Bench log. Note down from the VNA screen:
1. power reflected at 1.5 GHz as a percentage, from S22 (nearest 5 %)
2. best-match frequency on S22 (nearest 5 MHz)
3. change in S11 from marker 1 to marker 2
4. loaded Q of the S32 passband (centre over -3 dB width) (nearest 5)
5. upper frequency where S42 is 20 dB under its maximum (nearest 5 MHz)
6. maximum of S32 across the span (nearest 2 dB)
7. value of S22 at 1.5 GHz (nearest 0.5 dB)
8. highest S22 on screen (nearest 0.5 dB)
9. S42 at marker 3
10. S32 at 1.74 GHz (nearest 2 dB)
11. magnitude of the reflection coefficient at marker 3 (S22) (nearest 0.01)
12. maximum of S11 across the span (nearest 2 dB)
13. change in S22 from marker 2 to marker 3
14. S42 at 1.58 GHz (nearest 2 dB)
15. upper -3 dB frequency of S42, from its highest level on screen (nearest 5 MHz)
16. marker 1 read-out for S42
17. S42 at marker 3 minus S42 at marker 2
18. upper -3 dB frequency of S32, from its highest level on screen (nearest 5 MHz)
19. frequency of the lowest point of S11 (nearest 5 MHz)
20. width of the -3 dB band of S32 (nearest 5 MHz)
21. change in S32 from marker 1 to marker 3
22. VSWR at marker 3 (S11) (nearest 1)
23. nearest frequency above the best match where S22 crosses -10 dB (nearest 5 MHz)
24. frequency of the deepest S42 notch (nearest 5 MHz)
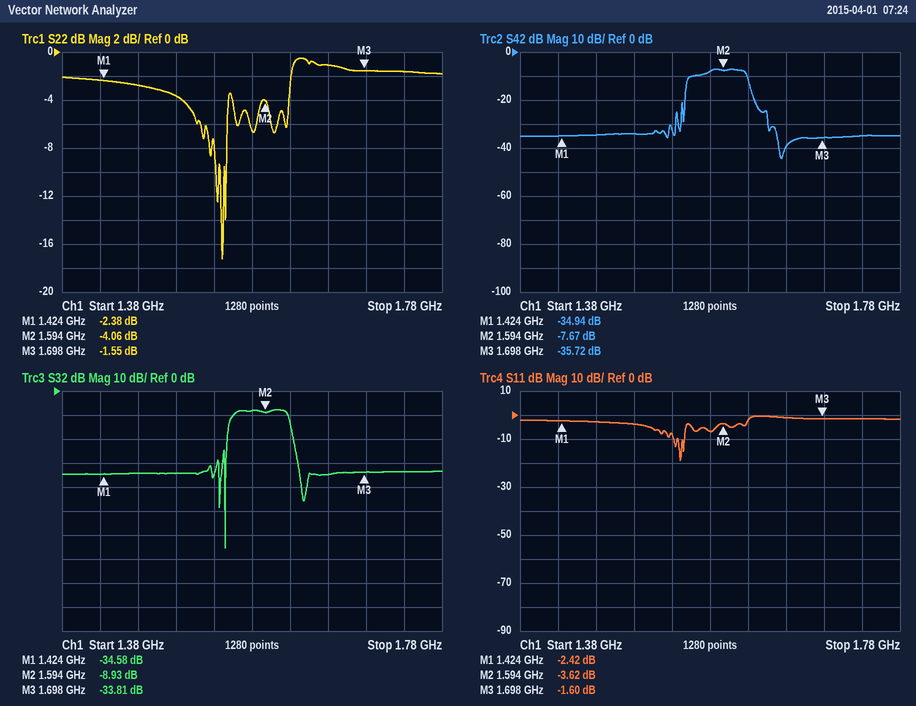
45 %
1.550 GHz
-1.20 dB
25
1.640 GHz
-8 dB
-3.5 dB
-0.5 dB
-35.72 dB
-34 dB
0.84
0 dB
2.51 dB
-8 dB
1.620 GHz
-34.94 dB
-28.05 dB
1.620 GHz
1.550 GHz
60 MHz
0.77 dB
11
1.550 GHz
1.655 GHz
